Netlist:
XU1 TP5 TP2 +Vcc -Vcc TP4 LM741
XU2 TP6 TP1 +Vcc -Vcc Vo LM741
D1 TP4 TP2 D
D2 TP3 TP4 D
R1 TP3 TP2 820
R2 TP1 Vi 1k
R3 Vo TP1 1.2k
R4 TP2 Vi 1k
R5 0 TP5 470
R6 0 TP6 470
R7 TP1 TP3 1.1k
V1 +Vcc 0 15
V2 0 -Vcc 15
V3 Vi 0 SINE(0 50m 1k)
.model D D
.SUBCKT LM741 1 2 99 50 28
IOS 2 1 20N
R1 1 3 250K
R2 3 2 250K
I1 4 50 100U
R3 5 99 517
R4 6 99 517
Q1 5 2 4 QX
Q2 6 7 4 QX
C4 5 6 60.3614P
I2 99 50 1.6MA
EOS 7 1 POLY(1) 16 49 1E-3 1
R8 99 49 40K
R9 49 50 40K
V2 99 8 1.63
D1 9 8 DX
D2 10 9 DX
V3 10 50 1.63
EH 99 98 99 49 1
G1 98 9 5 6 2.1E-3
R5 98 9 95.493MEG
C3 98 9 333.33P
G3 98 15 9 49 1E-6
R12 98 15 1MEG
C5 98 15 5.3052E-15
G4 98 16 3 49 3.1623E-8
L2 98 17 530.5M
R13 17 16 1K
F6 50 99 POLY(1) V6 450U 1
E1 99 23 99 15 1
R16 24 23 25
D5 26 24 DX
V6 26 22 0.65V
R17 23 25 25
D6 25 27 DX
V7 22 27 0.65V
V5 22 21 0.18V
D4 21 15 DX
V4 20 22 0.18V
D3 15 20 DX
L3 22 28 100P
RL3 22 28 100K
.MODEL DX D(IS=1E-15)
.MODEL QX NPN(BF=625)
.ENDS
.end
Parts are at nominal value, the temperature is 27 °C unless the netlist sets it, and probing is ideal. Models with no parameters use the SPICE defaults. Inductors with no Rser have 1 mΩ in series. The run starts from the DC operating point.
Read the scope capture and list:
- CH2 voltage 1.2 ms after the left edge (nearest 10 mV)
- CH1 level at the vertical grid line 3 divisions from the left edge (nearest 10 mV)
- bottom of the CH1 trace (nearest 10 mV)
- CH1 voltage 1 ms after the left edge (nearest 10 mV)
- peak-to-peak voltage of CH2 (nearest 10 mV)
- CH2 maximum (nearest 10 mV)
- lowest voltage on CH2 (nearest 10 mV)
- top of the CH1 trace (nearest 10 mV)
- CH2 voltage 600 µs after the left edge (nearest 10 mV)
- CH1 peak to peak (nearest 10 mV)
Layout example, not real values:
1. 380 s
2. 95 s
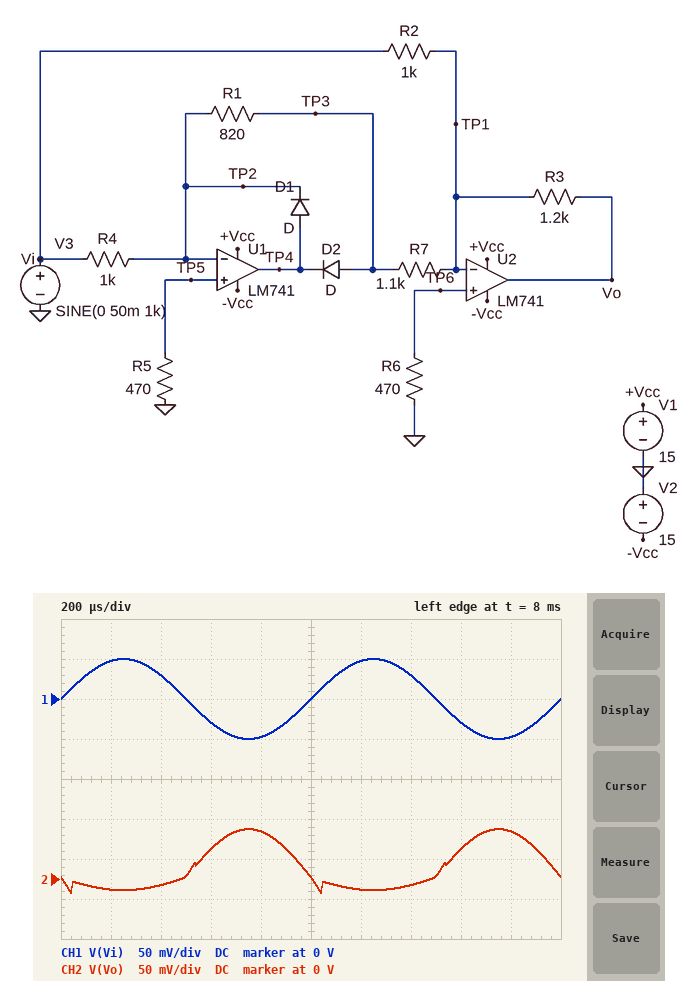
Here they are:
1. -10 mV
2. -30 mV
3. -50 mV
4. 0 V
5. 80 mV
6. 60 mV
7. -20 mV
8. 50 mV
9. 40 mV
10. 100 mV
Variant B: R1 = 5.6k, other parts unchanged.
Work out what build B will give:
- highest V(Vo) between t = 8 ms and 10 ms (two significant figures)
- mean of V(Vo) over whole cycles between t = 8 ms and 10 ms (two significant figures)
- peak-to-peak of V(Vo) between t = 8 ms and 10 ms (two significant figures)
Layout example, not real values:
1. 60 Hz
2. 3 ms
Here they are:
1. 240 mV
2. 95 mV
3. 250 mV
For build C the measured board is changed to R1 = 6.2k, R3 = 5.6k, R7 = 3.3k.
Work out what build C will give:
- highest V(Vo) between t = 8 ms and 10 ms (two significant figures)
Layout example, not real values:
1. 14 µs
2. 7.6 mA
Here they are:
1. 290 mV
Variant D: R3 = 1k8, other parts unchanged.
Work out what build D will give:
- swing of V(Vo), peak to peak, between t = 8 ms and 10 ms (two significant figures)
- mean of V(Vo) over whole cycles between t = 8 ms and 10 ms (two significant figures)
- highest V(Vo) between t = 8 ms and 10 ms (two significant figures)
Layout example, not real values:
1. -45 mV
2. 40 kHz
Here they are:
1. 120 mV
2. 23 mV
3. 93 mV
